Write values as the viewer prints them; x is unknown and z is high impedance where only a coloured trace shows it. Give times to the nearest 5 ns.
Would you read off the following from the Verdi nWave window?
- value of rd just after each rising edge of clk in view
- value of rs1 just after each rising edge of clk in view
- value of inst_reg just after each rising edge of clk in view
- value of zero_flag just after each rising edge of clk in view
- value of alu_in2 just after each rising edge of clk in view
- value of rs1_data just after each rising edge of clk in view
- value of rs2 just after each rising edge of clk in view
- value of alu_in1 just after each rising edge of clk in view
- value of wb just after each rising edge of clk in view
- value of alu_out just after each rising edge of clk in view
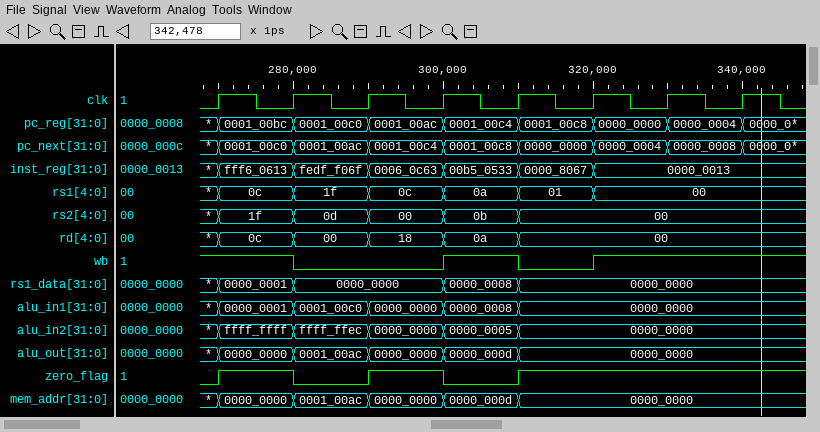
0c, 00, 18, 0a, 00, 00, 00, 00
0c, 1f, 0c, 0a, 01, 00, 00, 00
fff6_0613, fedf_f06f, 0006_0c63, 00b5_0533, 0000_8067, 0000_0013, 0000_0013, 0000_0013
1 0 1 0 1 1 1 1
ffff_ffff, ffff_ffec, 0000_0000, 0000_0005, 0000_0000, 0000_0000, 0000_0000, 0000_0000
0000_0001, 0000_0000, 0000_0000, 0000_0008, 0000_0000, 0000_0000, 0000_0000, 0000_0000
1f, 0d, 00, 0b, 00, 00, 00, 00
0000_0001, 0001_00c0, 0000_0000, 0000_0008, 0000_0000, 0000_0000, 0000_0000, 0000_0000
1 0 0 1 0 1 1 1
0000_0000, 0001_00ac, 0000_0000, 0000_000d, 0000_0000, 0000_0000, 0000_0000, 0000_0000
